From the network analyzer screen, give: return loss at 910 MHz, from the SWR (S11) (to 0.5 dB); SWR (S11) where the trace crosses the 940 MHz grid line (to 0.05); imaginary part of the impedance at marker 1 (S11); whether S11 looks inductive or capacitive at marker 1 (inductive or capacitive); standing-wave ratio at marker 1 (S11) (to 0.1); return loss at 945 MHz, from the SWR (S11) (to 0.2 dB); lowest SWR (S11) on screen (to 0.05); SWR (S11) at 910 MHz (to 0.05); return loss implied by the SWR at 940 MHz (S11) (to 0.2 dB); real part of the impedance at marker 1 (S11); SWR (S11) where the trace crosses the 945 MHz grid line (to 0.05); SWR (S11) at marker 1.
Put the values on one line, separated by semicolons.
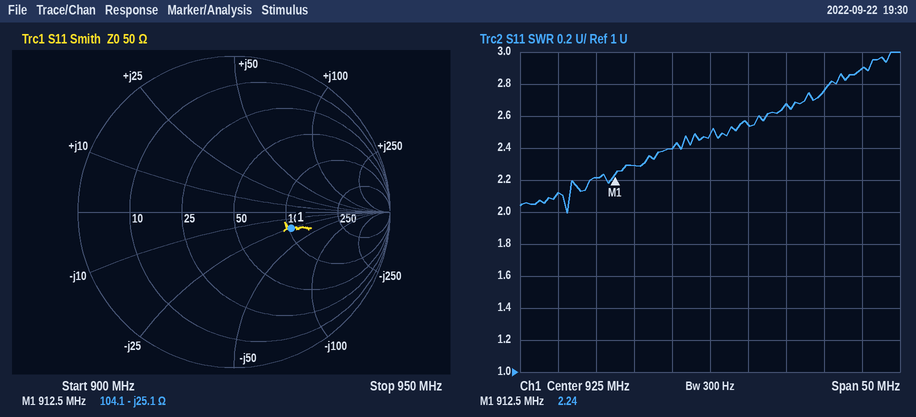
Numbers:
8.5 dB; 2.75; -25.1 Ω; capacitive; 2.2; 6.2 dB; 2.00; 2.20; 6.6 dB; 104.1 Ω; 2.90; 2.24
